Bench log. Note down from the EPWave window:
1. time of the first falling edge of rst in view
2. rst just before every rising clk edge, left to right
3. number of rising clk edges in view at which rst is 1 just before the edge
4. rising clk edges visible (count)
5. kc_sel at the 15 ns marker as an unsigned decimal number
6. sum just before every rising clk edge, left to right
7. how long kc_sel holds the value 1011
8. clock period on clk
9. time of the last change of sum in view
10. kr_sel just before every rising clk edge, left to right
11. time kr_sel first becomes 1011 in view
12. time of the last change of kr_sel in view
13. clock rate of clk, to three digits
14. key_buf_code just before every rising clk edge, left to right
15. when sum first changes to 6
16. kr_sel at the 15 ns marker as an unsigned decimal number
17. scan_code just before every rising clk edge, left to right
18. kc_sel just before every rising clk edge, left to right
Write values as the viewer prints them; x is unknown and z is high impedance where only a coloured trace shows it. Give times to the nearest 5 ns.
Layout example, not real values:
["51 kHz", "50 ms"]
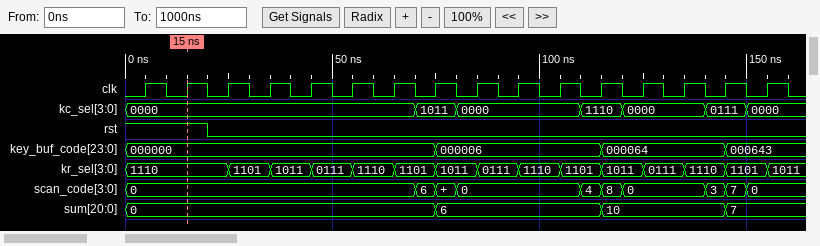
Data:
["20 ns", "1 1 0 0 0 0 0 0 0 0 0 0 0 0 0 0", "2", "16", "0", "0, 0, 0, 0, 0, 0, 0, 0, 6, 6, 6, 6, 10, 10, 10, 7", "10 ns", "10 ns", "145 ns", "1110, 1110, 1110, 1101, 1011, 0111, 1110, 1101, 1011, 0111, 1110, 1101, 1011, 0111, 1110, 1101", "35 ns", "155 ns", "100 MHz", "000000, 000000, 000000, 000000, 000000, 000000, 000000, 000000, 000006, 000006, 000006, 000006, 000064, 000064, 000064, 000643", "75 ns", "14", "0, 0, 0, 0, 0, 0, 0, 6, 0, 0, 0, 4, 0, 0, 3, 0", "0000, 0000, 0000, 0000, 0000, 0000, 0000, 1011, 0000, 0000, 0000, 1110, 0000, 0000, 0111, 0000"]
